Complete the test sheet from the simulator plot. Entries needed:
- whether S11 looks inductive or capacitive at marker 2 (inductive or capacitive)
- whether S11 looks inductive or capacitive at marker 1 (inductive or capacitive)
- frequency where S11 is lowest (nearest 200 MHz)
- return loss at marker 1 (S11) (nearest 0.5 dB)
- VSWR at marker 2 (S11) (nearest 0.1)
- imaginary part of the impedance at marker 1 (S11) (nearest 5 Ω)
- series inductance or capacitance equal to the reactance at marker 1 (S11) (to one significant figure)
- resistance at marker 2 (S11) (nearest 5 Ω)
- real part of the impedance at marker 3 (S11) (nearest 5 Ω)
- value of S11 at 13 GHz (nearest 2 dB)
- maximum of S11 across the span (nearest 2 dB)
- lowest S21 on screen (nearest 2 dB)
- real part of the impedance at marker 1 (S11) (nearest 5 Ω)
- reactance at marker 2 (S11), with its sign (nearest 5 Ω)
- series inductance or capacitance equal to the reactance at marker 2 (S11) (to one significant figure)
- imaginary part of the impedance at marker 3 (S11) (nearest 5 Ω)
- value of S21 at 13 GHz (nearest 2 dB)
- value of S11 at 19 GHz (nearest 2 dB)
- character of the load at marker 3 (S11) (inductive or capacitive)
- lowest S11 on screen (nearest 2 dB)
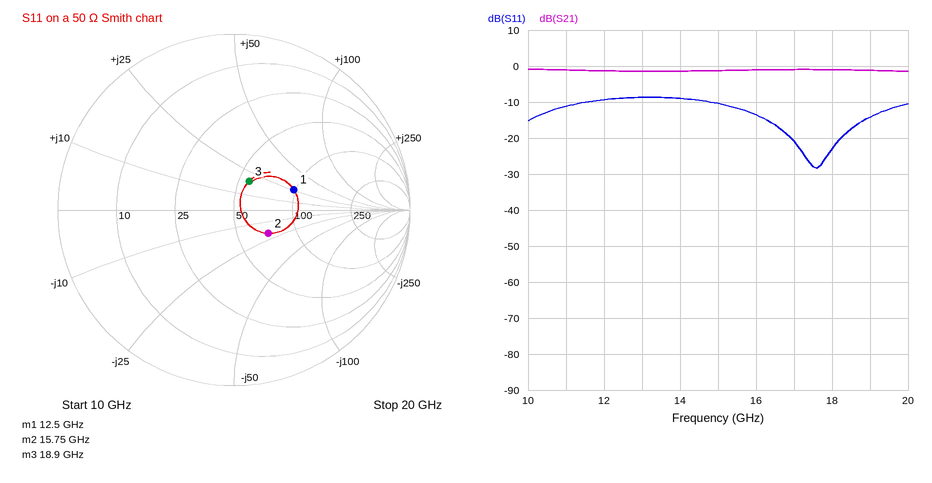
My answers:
capacitive
inductive
17.6 GHz
9.0 dB
1.6
+25 Ω
300 pH
70 Ω
55 Ω
-8 dB
-8 dB
-2 dB
95 Ω
-20 Ω
500 fF
+20 Ω
-2 dB
-14 dB
inductive
-28 dB
